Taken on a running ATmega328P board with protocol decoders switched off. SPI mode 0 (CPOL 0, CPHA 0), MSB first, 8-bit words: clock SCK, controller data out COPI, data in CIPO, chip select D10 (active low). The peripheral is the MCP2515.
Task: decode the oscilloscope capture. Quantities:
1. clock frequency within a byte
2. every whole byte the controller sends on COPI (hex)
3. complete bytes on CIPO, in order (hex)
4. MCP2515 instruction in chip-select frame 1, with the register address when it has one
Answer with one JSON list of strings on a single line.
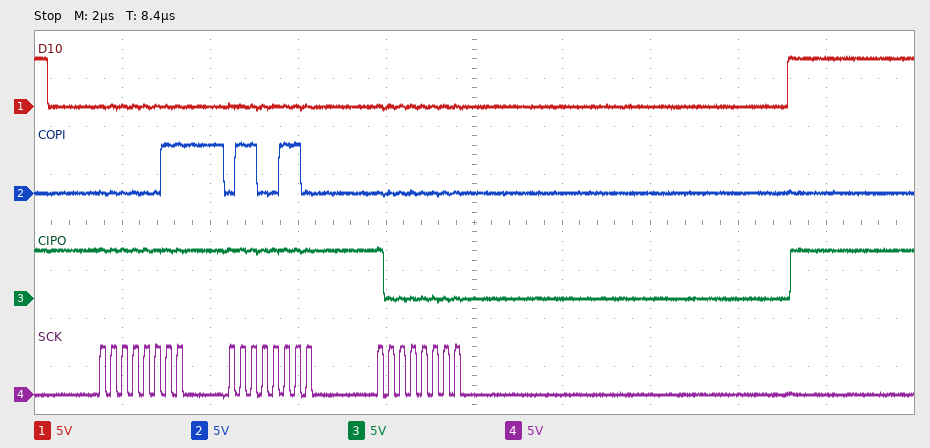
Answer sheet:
["4 MHz", "03 66 00", "FF FF 80", "READ 0x66"]
